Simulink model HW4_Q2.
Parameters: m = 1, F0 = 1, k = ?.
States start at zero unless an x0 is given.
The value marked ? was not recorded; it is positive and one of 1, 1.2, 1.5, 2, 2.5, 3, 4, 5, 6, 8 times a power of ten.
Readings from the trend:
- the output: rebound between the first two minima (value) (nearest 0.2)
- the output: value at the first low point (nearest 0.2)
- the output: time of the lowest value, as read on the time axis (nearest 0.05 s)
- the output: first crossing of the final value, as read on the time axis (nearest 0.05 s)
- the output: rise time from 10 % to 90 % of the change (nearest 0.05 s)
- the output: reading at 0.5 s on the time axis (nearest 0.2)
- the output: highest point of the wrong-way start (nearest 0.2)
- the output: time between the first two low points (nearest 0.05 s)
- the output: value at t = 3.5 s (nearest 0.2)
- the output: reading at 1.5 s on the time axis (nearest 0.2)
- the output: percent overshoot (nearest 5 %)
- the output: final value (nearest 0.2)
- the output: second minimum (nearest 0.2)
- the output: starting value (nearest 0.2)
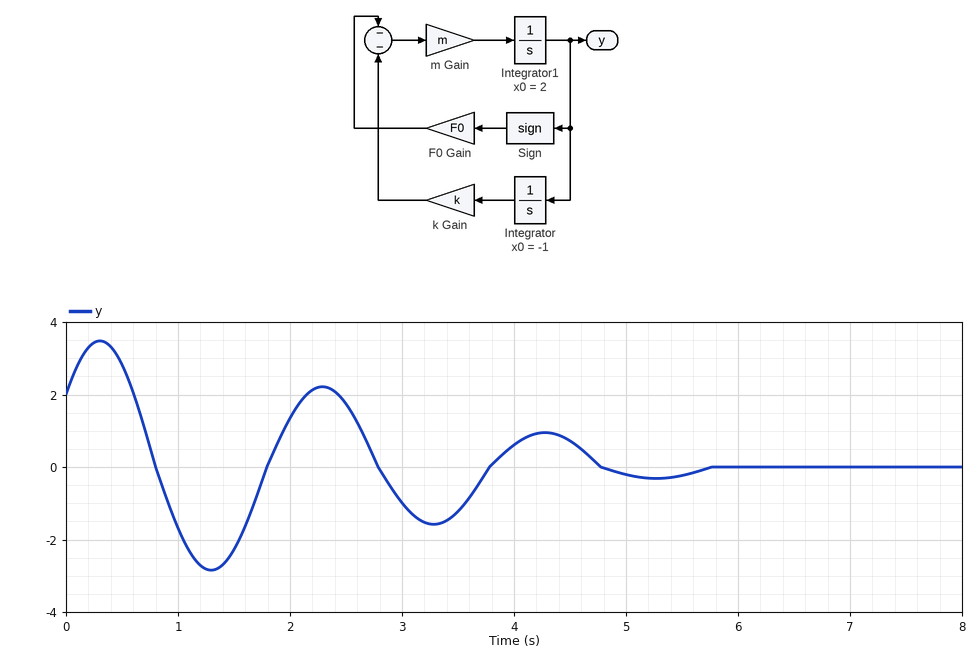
2.2
-2.8
1.30 s
0.80 s
0.15 s
2.8
3.4
2.00 s
-1.2
-2.2
145 %
0.0
-1.6
2.0
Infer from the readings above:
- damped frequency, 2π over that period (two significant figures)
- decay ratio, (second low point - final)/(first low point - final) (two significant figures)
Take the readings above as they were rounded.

3.1 rad/s
0.57
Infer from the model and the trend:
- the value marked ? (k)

10
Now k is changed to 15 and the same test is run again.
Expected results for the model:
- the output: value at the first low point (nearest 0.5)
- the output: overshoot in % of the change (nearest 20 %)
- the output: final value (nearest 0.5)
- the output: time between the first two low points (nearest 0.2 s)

-3.5
180 %
0.0
1.6 s
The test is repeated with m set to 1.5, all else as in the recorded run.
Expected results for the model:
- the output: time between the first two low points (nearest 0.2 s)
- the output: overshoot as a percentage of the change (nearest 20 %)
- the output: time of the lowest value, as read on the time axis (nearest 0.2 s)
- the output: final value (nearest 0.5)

1.6 s
160 %
1.0 s
0.0
